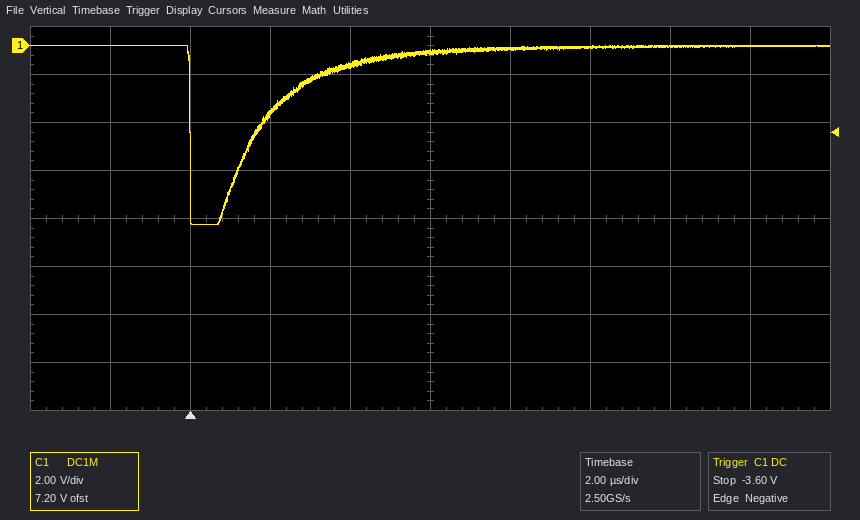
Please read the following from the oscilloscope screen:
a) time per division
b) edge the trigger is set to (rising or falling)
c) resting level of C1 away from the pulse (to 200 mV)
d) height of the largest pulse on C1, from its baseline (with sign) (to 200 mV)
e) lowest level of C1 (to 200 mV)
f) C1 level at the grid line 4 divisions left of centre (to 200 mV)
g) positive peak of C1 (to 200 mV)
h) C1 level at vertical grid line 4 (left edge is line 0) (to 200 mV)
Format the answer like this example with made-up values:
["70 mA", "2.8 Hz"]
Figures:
["2 µs", "falling", "0.0 V", "-7.4 V", "-7.4 V", "0.0 V", "0.0 V", "-800 mV"]
